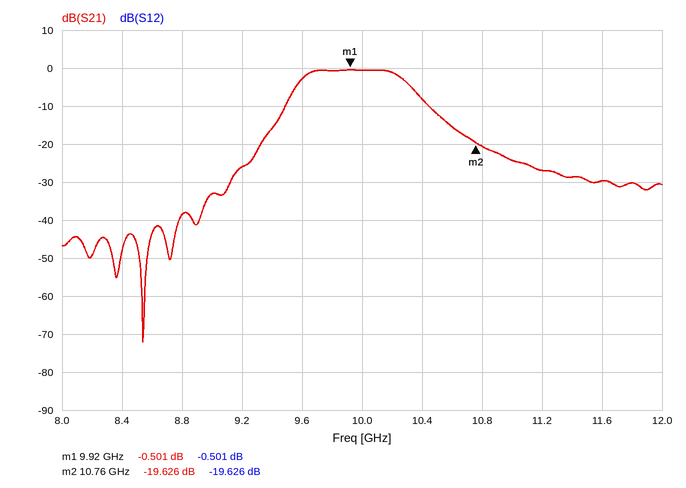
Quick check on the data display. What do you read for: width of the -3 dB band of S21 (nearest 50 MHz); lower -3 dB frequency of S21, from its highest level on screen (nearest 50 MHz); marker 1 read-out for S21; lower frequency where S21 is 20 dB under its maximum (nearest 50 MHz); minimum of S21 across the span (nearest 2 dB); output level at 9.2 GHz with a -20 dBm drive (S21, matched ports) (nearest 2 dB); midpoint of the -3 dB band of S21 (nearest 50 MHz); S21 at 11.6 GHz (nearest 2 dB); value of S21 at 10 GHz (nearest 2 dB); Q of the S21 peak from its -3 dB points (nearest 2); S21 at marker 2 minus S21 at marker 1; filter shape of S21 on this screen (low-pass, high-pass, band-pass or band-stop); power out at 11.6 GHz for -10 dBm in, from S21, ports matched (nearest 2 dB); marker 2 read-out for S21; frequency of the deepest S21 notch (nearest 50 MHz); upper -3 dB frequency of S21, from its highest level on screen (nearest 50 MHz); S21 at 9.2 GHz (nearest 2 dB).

700 MHz
9.60 GHz
-0.501 dB
9.30 GHz
-72 dB
-46 dBm
9.95 GHz
-30 dB
0 dB
14
-19.125 dB
band-pass
-40 dBm
-19.626 dB
8.55 GHz
10.30 GHz
-26 dB
